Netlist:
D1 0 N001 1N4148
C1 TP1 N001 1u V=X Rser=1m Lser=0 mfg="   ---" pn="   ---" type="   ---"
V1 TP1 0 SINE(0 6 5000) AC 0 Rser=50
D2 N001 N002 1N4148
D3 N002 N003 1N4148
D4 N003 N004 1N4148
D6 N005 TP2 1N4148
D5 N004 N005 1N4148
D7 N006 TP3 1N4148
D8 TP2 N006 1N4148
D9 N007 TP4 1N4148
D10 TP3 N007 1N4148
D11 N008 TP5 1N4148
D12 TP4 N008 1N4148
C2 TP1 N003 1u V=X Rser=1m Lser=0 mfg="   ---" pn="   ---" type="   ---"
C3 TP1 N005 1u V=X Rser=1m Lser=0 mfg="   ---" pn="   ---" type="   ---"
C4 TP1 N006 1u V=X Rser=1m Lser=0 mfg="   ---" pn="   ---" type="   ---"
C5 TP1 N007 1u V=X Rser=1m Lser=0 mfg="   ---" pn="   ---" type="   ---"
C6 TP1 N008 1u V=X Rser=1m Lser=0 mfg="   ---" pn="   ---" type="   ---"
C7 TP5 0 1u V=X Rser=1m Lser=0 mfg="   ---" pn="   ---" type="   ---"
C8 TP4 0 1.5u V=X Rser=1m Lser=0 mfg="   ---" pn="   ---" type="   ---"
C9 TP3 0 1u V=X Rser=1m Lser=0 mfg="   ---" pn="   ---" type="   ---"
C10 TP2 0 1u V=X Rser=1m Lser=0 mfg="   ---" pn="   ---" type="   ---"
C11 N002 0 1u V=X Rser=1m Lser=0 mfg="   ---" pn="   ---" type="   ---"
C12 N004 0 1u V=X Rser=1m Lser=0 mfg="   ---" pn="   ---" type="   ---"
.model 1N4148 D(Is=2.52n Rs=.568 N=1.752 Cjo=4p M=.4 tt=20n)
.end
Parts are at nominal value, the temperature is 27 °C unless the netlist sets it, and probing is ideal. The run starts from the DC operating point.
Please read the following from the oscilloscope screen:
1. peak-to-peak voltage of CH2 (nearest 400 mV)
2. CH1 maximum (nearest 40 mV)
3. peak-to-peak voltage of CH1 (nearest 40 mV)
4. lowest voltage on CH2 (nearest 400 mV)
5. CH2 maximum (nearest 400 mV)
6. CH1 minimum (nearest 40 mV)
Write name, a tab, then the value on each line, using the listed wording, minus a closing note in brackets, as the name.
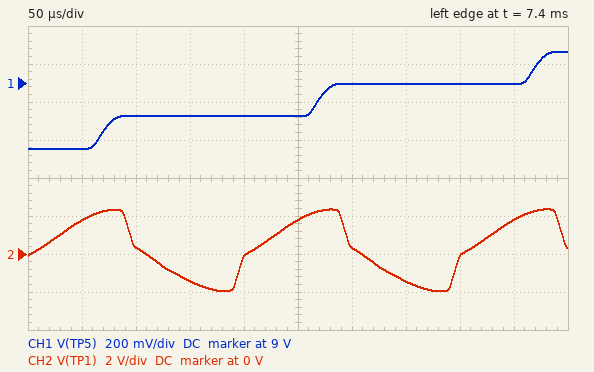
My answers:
peak-to-peak voltage of CH2	4.4 V
CH1 maximum	9.16 V
peak-to-peak voltage of CH1	520 mV
lowest voltage on CH2	-2.0 V
CH2 maximum	2.4 V
CH1 minimum	8.64 V
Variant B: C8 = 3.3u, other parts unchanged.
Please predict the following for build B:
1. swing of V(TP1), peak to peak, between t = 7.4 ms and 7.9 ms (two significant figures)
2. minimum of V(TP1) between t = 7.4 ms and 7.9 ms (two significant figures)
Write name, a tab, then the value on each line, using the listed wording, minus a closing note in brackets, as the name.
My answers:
swing of V(TP1), peak to peak, between t = 7.4 ms and 7.9 ms	4.1 V
minimum of V(TP1) between t = 7.4 ms and 7.9 ms	-1.9 V
